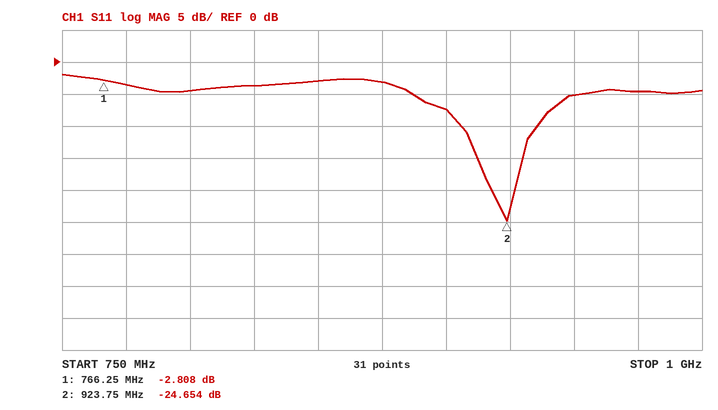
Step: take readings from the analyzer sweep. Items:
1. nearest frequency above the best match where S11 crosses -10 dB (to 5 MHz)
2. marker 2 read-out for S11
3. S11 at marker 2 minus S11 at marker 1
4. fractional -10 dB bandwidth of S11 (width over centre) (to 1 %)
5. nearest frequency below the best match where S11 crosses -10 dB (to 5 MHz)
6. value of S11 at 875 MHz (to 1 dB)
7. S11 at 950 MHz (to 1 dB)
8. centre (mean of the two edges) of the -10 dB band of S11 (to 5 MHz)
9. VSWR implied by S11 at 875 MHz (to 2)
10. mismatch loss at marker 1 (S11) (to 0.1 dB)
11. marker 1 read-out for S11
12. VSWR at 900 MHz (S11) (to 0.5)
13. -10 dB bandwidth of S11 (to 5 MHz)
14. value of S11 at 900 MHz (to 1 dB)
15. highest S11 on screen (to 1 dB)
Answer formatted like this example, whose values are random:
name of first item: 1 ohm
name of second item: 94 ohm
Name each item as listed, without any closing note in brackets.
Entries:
nearest frequency above the best match where S11 crosses -10 dB: 935 MHz
marker 2 read-out for S11: -24.654 dB
S11 at marker 2 minus S11 at marker 1: -21.846 dB
fractional -10 dB bandwidth of S11 (width over centre): 3 %
nearest frequency below the best match where S11 crosses -10 dB: 905 MHz
value of S11 at 875 MHz: -3 dB
S11 at 950 MHz: -5 dB
centre (mean of the two edges) of the -10 dB band of S11: 920 MHz
VSWR implied by S11 at 875 MHz: 6
mismatch loss at marker 1 (S11): 3.2 dB
marker 1 read-out for S11: -2.808 dB
VSWR at 900 MHz (S11): 2.5
-10 dB bandwidth of S11: 30 MHz
value of S11 at 900 MHz: -7 dB
highest S11 on screen: -2 dB
